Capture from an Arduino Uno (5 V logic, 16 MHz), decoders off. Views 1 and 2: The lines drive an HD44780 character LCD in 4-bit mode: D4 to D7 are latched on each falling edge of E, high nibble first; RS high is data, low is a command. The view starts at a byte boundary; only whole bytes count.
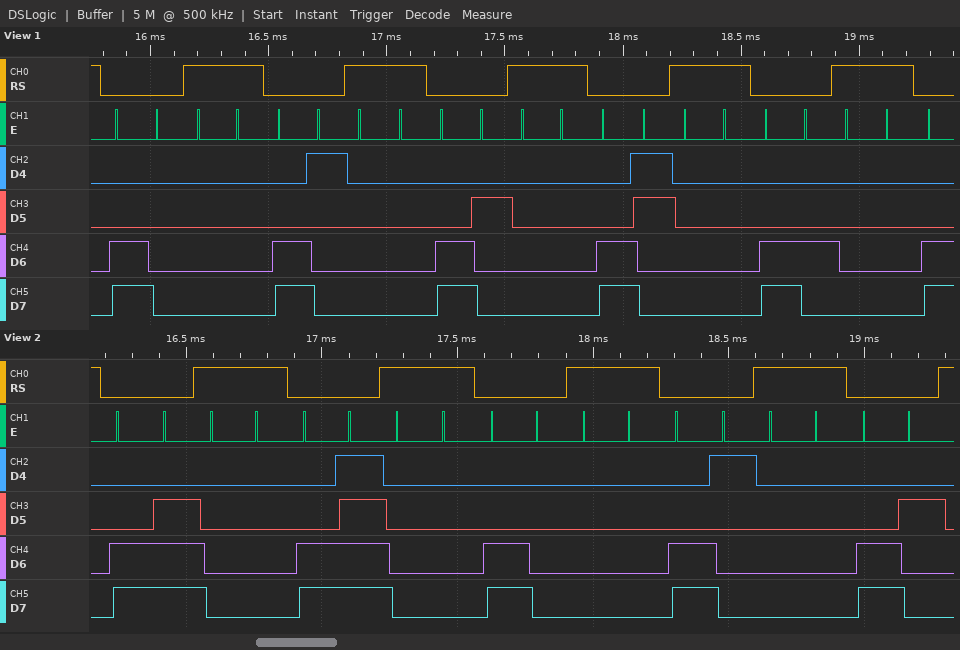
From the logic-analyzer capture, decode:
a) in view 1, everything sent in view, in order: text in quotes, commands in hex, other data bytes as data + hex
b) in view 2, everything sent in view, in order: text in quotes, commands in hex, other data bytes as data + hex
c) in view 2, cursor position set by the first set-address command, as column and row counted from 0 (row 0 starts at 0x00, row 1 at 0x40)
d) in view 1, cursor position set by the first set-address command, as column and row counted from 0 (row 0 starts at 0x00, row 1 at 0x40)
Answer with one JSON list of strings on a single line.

["0xC0 data 00 0xC1 data 00 0xC2 data 00 0xC3 data 00 0xC4 data 00", "0xCE data 00 0xCF data 00 0xC0 data 00 0xC1 data 00 0xC2", "column 14, row 1", "column 0, row 1"]
